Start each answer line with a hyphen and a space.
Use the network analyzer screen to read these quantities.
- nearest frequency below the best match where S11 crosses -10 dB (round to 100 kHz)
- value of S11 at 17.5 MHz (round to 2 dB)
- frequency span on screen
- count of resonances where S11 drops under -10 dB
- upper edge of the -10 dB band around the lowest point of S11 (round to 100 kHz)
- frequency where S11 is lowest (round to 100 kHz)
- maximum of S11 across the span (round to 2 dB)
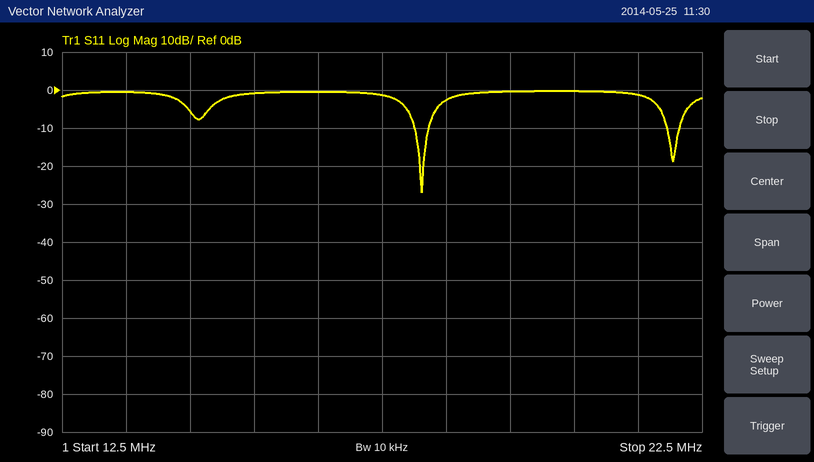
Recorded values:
- 18.0 MHz
- -2 dB
- 10 MHz
- 2
- 18.2 MHz
- 18.1 MHz
- 0 dB
